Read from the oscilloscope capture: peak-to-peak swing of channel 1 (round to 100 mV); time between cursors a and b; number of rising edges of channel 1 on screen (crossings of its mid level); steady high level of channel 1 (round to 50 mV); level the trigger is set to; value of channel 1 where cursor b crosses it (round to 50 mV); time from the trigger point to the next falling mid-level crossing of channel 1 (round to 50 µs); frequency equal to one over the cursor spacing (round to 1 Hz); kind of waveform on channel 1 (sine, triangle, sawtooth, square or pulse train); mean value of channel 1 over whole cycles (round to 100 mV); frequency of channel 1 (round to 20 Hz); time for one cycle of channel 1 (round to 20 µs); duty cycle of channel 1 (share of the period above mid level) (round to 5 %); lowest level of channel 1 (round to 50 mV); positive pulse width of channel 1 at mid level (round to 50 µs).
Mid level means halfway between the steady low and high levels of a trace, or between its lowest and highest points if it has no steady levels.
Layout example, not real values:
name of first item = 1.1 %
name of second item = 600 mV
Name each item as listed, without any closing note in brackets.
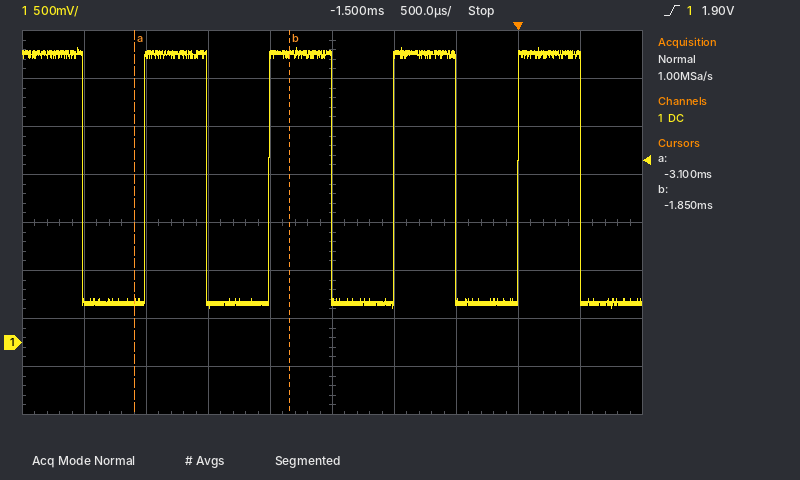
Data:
peak-to-peak swing of channel 1 = 2.70 V
time between cursors a and b = 1.25 ms
number of rising edges of channel 1 on screen = 4
steady high level of channel 1 = 3.00 V
level the trigger is set to = 1.90 V
value of channel 1 where cursor b crosses it = 3.00 V
time from the trigger point to the next falling mid-level crossing of channel 1 = 500 µs
frequency equal to one over the cursor spacing = 800 Hz
kind of waveform on channel 1 = square
mean value of channel 1 over whole cycles = 1.7 V
frequency of channel 1 = 1.00 kHz
time for one cycle of channel 1 = 1.00 ms
duty cycle of channel 1 (share of the period above mid level) = 50 %
lowest level of channel 1 = 350 mV
positive pulse width of channel 1 at mid level = 500 µs
